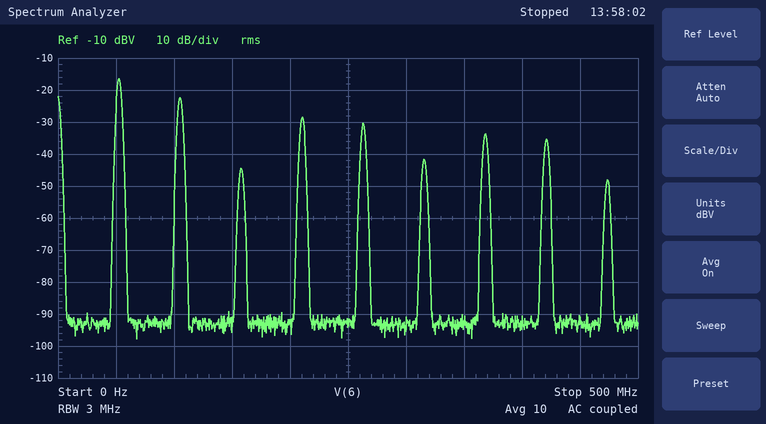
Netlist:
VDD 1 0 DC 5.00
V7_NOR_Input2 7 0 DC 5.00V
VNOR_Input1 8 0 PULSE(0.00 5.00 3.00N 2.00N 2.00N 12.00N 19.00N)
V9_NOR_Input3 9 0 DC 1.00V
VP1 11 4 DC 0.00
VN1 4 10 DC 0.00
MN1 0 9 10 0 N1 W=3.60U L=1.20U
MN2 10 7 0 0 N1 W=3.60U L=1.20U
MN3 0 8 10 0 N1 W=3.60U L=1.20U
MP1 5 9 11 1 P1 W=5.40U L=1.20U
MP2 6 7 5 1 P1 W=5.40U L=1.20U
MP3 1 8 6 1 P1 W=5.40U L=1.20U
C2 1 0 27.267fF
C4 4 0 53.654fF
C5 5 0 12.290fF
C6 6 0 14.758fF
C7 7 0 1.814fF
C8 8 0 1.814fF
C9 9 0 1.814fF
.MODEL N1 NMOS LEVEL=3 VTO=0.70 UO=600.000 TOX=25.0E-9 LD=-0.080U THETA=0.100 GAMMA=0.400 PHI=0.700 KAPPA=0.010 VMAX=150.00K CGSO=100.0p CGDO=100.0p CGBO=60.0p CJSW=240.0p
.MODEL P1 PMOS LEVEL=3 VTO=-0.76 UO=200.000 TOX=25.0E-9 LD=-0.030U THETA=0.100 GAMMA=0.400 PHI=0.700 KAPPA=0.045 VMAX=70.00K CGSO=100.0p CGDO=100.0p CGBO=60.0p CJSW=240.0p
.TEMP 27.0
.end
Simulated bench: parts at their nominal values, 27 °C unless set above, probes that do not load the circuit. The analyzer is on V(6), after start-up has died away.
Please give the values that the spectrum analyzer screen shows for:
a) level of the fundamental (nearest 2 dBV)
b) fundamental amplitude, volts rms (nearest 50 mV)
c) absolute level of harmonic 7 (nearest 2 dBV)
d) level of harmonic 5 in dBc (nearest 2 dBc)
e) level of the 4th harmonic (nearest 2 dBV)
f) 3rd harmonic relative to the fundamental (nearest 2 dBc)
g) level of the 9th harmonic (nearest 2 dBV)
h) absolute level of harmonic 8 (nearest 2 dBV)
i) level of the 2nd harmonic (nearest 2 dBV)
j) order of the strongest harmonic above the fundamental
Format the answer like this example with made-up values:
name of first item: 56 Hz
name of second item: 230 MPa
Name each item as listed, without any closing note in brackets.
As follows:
level of the fundamental: -16 dBV
fundamental amplitude, volts rms: 150 mV
absolute level of harmonic 7: -34 dBV
level of harmonic 5 in dBc: -14 dBc
level of the 4th harmonic: -28 dBV
3rd harmonic relative to the fundamental: -28 dBc
level of the 9th harmonic: -48 dBV
absolute level of harmonic 8: -36 dBV
level of the 2nd harmonic: -22 dBV
order of the strongest harmonic above the fundamental: 2
